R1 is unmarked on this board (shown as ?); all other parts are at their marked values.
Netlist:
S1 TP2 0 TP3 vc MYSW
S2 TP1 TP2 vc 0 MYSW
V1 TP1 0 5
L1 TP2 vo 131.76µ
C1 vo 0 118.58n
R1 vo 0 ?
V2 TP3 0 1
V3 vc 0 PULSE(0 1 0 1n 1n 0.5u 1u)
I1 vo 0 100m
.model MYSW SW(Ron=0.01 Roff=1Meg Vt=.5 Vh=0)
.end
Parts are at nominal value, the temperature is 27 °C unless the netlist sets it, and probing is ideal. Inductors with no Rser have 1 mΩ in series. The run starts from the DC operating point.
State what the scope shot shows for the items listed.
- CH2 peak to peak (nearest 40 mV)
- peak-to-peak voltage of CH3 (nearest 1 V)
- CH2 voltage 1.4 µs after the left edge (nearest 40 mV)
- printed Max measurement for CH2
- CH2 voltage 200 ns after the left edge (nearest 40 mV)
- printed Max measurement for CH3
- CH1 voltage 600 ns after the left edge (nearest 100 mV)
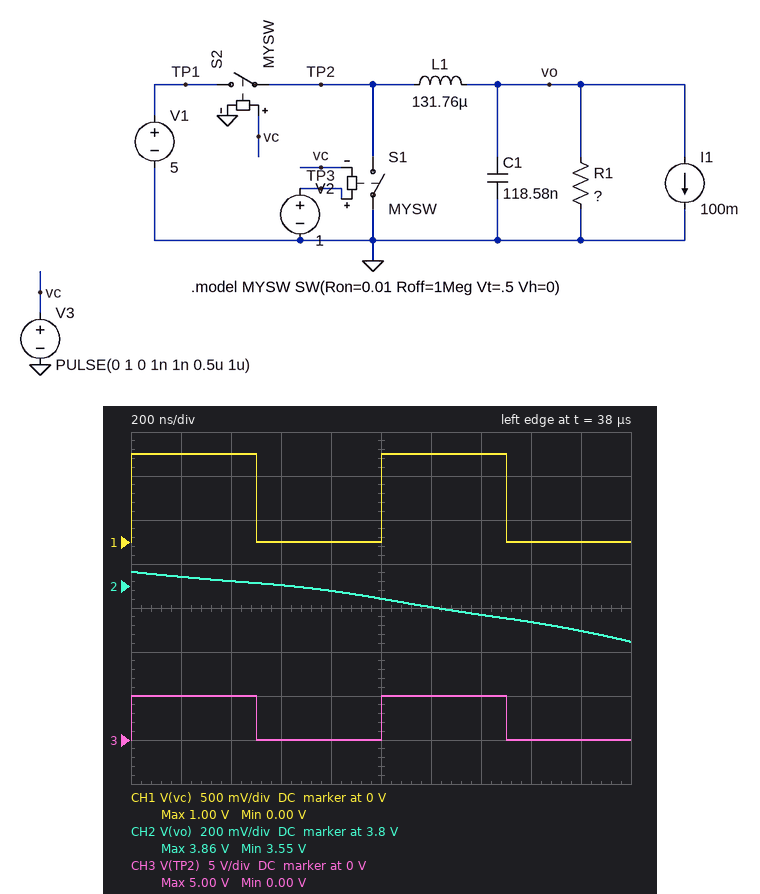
320 mV
5 V
3.68 V
3.86 V
3.84 V
5.00 V
0 V
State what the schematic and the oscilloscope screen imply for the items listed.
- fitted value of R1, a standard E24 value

270 Ω
